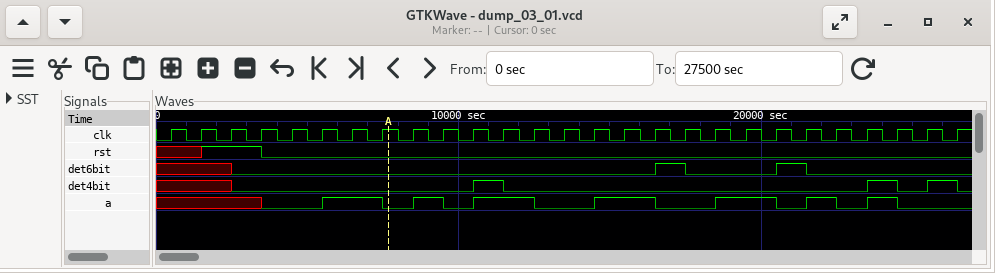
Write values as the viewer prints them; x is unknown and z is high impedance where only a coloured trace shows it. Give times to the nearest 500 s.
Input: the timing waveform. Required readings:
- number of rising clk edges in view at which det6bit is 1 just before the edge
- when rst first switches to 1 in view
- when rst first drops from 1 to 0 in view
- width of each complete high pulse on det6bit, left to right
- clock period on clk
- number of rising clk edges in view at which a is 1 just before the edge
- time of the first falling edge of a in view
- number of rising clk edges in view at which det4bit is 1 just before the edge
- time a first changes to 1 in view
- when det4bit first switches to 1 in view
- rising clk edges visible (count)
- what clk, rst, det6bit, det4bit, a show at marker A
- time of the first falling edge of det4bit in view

2
1500 s
3500 s
1000 s, 1000 s
1000 s
11
7500 s
3
5500 s
10500 s
27
clk=1, rst=0, det6bit=0, det4bit=0, a=0
11500 s
